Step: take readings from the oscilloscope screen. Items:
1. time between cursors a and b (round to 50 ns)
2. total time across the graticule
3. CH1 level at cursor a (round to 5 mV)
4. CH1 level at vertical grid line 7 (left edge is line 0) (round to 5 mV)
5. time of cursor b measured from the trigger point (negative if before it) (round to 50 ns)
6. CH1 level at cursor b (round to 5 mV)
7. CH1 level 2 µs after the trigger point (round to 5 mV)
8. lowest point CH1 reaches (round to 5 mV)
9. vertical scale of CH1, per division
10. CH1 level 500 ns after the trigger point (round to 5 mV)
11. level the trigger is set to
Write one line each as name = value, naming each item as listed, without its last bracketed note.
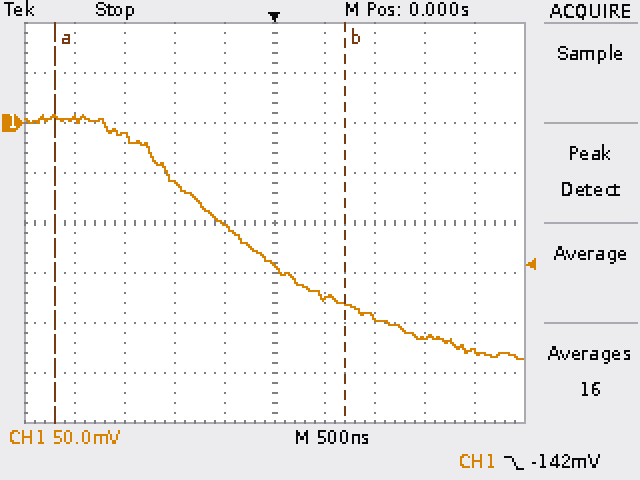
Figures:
time between cursors a and b = 2.90 µs
total time across the graticule = 5 µs
CH1 level at cursor a = 5 mV
CH1 level at vertical grid line 7 (left edge is line 0) = -195 mV
time of cursor b measured from the trigger point (negative if before it) = +700 ns
CH1 level at cursor b = -180 mV
CH1 level 2 µs after the trigger point = -230 mV
lowest point CH1 reaches = -235 mV
vertical scale of CH1, per division = 50 mV
CH1 level 500 ns after the trigger point = -175 mV
level the trigger is set to = -142 mV
